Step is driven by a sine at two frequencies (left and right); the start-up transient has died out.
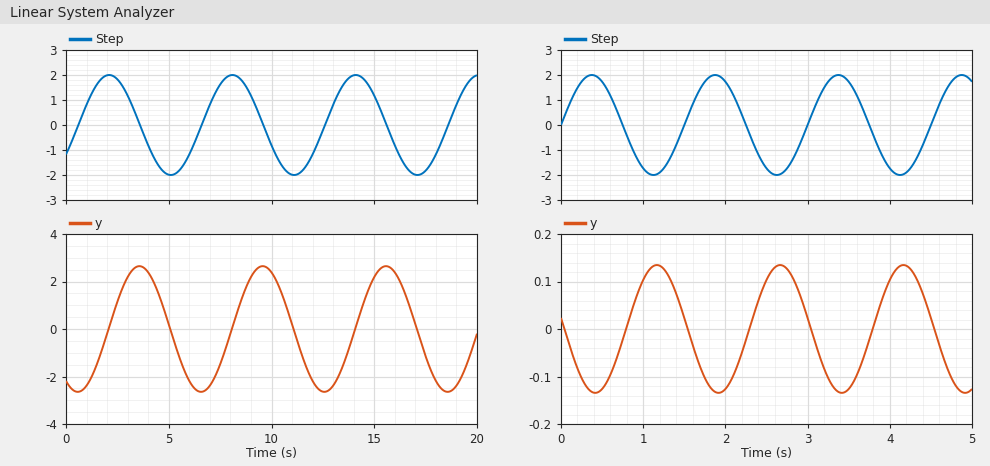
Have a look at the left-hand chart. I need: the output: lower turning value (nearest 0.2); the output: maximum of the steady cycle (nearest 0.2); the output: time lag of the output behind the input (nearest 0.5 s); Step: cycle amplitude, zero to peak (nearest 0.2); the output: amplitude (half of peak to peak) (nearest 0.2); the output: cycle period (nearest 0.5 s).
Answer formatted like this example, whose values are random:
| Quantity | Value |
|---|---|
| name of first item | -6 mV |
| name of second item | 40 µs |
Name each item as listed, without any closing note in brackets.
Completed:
| Quantity | Value |
|---|---|
| the output: lower turning value | -2.6 |
| the output: maximum of the steady cycle | 2.6 |
| the output: time lag of the output behind the input | 1.5 s |
| Step: cycle amplitude, zero to peak | 2.0 |
| the output: amplitude (half of peak to peak) | 2.6 |
| the output: cycle period | 6.0 s |
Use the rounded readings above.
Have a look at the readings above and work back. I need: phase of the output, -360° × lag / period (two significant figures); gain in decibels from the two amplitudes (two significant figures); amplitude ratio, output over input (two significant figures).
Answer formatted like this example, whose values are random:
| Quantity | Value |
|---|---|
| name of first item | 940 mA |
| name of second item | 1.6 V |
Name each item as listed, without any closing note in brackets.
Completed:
| Quantity | Value |
|---|---|
| phase of the output, -360° × lag / period | -90° |
| gain in decibels from the two amplitudes | 2.3 dB |
| amplitude ratio, output over input | 1.3 |
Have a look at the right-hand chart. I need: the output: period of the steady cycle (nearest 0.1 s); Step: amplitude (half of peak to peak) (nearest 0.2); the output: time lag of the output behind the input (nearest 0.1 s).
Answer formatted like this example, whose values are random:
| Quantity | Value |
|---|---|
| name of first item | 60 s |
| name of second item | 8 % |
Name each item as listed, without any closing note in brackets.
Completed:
| Quantity | Value |
|---|---|
| the output: period of the steady cycle | 1.5 s |
| Step: amplitude (half of peak to peak) | 2.0 |
| the output: time lag of the output behind the input | 0.8 s |
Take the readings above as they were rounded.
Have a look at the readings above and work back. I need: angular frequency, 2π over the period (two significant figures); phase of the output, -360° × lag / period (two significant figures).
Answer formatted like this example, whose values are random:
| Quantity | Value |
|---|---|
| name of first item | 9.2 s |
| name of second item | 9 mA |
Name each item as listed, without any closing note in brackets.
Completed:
| Quantity | Value |
|---|---|
| angular frequency, 2π over the period | 4.2 rad/s |
| phase of the output, -360° × lag / period | -190° |
